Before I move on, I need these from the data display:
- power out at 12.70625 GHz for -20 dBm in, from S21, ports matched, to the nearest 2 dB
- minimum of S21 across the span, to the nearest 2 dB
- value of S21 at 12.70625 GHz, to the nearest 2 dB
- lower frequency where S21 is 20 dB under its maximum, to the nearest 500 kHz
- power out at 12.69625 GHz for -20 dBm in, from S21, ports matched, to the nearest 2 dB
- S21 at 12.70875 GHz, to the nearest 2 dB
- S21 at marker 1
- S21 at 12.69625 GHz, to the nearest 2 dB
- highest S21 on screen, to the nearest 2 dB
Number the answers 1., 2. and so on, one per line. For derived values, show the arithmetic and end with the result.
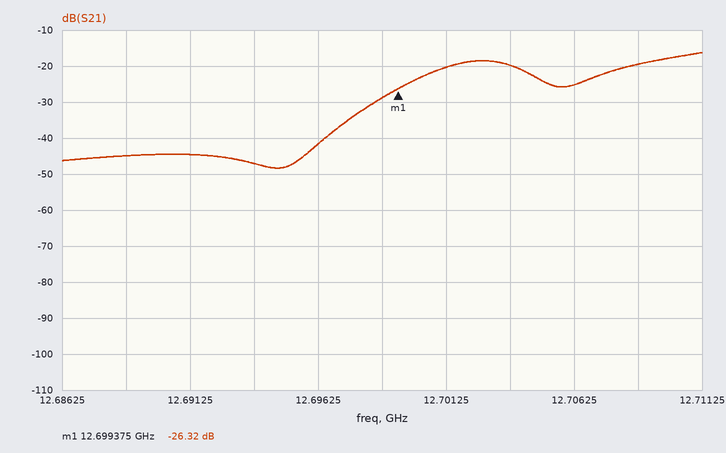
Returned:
1. -20 dBm + (-26 dB) = -46 dBm
2. -48 dB
3. -26 dB
4. 12.6970 GHz
5. -20 dBm + (-42 dB) = -62 dBm
6. -20 dB
7. -26.32 dB
8. -42 dB
9. -16 dB
